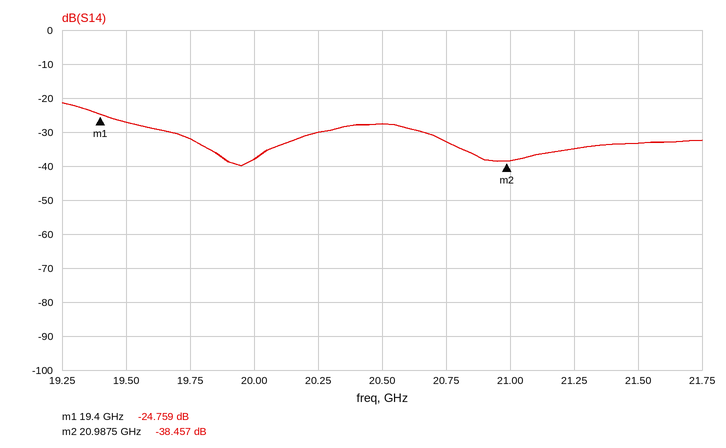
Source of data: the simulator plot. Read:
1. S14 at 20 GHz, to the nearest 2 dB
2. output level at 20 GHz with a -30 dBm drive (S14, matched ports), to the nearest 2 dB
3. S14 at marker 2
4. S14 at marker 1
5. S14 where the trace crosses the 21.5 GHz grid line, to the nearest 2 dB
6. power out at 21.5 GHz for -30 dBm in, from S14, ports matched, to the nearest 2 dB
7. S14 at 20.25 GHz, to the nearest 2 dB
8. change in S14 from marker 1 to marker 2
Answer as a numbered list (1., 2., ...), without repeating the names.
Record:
1. -38 dB
2. -68 dBm
3. -38.457 dB
4. -24.759 dB
5. -34 dB
6. -64 dBm
7. -30 dB
8. -13.698 dB
